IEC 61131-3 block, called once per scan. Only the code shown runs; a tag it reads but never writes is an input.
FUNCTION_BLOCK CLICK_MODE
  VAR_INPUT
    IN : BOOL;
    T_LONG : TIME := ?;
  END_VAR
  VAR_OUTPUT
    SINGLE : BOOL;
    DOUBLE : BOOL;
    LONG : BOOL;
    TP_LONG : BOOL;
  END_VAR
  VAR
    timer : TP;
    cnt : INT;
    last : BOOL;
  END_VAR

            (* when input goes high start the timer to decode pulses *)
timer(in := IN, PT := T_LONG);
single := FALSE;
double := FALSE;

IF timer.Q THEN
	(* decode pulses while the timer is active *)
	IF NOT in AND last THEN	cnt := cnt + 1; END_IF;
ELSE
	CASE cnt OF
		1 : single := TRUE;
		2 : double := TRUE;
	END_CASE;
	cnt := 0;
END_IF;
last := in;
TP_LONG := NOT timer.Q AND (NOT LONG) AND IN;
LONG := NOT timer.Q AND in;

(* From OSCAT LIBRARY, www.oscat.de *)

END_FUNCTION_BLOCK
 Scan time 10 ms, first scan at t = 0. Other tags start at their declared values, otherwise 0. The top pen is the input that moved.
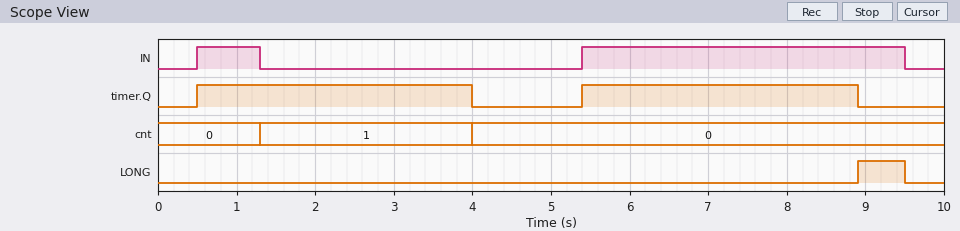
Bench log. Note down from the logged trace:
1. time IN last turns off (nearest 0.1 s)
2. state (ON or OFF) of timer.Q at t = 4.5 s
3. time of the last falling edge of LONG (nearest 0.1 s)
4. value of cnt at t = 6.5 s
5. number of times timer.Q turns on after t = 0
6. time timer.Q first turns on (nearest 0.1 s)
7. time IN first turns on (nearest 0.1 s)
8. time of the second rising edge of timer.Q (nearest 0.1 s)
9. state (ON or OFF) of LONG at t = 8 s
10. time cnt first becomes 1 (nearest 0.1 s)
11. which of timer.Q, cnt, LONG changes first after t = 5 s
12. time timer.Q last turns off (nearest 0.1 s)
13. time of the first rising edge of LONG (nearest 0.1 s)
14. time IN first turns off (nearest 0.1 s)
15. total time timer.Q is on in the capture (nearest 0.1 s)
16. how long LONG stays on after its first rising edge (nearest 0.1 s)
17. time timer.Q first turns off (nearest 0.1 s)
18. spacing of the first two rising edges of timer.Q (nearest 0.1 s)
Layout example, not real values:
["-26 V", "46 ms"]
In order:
["9.5 s", "OFF", "9.5 s", "0", "2", "0.5 s", "0.5 s", "5.4 s", "OFF", "1.3 s", "timer.Q", "8.9 s", "8.9 s", "1.3 s", "7.0 s", "0.6 s", "4.0 s", "4.9 s"]
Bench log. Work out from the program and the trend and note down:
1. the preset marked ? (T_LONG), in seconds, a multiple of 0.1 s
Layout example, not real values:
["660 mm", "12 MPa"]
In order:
["3.5 s"]
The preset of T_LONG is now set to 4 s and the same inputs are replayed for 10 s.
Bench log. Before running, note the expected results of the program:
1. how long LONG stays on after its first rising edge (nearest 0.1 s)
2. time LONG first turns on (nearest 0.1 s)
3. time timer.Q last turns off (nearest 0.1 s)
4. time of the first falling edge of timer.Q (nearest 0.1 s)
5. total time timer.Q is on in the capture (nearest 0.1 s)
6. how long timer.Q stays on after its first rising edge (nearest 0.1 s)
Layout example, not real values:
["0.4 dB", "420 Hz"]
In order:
["0.1 s", "9.4 s", "9.4 s", "4.5 s", "8.0 s", "4.0 s"]
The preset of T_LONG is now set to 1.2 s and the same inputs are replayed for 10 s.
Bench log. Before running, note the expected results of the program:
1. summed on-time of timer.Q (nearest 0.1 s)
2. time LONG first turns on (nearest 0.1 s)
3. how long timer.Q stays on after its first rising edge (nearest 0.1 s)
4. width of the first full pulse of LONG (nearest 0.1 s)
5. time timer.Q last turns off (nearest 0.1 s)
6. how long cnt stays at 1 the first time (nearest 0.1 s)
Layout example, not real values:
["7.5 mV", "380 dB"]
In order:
["2.4 s", "6.6 s", "1.2 s", "2.9 s", "6.6 s", "0.4 s"]
